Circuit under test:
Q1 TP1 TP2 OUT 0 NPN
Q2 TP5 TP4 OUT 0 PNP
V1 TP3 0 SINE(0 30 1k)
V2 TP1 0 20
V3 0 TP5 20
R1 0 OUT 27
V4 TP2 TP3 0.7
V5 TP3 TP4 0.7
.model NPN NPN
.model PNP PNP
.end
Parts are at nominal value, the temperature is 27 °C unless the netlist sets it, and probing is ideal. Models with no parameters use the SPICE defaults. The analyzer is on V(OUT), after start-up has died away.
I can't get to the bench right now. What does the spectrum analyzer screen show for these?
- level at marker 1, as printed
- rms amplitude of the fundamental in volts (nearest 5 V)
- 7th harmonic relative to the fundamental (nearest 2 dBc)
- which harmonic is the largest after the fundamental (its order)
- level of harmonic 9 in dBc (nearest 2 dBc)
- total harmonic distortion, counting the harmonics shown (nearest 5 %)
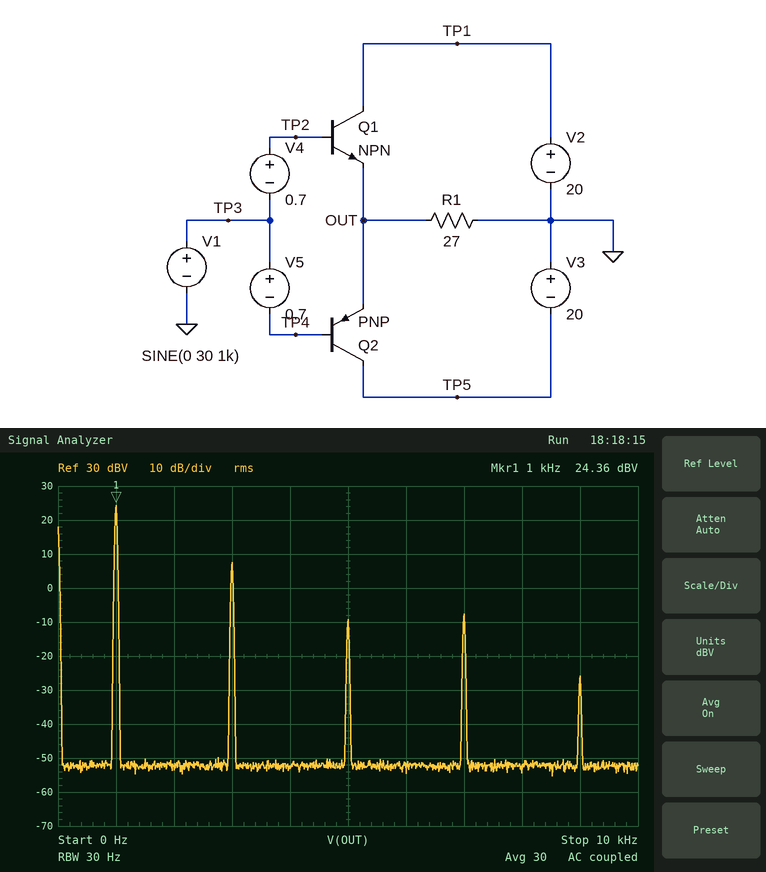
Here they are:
24.36 dBV
15 V
-32 dBc
3
-50 dBc
15 %
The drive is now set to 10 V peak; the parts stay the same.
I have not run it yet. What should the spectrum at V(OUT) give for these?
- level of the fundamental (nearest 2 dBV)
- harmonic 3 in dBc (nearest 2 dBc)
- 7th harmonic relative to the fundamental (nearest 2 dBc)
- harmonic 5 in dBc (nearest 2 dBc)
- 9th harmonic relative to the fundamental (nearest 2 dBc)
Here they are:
16 dBV
-42 dBc
-50 dBc
-48 dBc
-54 dBc
